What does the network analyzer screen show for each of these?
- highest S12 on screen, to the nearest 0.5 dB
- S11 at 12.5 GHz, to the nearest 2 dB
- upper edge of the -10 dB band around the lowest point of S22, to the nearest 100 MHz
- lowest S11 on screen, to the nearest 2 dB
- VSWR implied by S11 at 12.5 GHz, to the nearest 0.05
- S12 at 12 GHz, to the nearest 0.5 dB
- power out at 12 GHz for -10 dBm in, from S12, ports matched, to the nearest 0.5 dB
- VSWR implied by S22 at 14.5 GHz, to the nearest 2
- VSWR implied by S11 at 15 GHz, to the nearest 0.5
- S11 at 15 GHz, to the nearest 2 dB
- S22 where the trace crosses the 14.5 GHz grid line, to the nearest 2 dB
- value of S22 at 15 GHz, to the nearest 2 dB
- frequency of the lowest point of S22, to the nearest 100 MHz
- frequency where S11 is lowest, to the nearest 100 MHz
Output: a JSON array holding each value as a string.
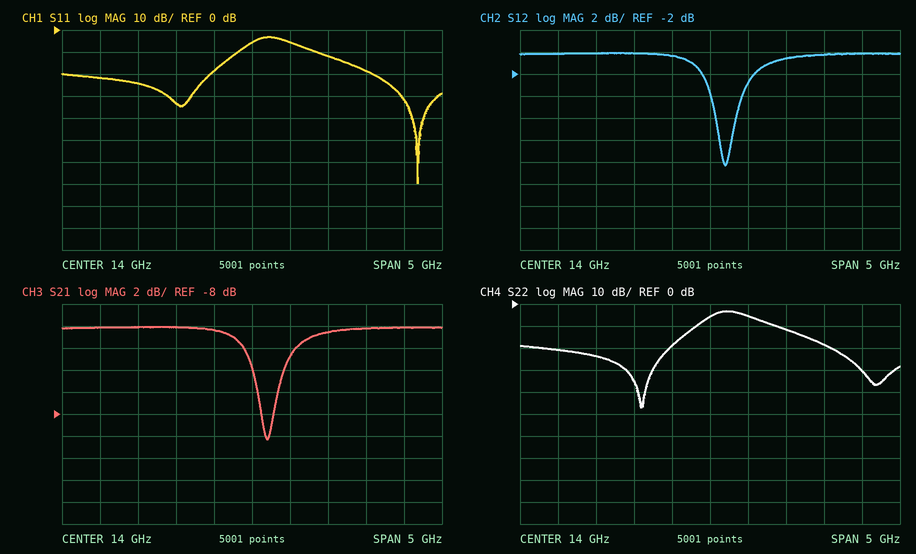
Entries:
["0.0 dB", "-24 dB", "13.8 GHz", "-70 dB", "1.15", "0.0 dB", "-10.0 dBm", "4", "1.5", "-12 dB", "-6 dB", "-12 dB", "13.1 GHz", "16.2 GHz"]
